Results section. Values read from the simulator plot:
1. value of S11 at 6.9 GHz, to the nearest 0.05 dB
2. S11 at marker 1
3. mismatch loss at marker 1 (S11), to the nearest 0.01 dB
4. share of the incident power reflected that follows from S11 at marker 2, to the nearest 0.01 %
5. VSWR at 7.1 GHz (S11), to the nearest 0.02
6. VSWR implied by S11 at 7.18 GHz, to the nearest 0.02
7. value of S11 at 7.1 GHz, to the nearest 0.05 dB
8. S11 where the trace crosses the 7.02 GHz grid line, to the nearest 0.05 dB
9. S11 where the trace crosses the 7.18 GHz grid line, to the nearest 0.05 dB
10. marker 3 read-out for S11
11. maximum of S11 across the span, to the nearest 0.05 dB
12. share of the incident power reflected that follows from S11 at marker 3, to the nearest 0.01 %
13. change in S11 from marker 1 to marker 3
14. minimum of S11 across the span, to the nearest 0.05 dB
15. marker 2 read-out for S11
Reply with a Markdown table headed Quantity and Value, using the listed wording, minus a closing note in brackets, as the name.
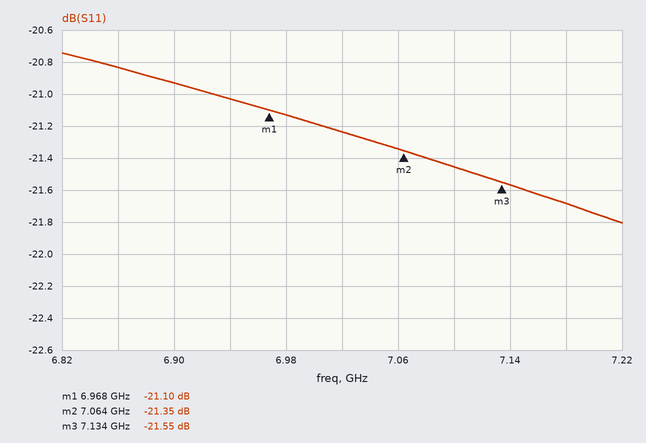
| Quantity | Value |
|---|---|
| value of S11 at 6.9 GHz, to the nearest 0.05 dB | -20.95 dB |
| S11 at marker 1 | -21.10 dB |
| mismatch loss at marker 1 (S11), to the nearest 0.01 dB | 0.03 dB |
| share of the incident power reflected that follows from S11 at marker 2, to the nearest 0.01 % | 0.73 % |
| VSWR at 7.1 GHz (S11), to the nearest 0.02 | 1.18 |
| VSWR implied by S11 at 7.18 GHz, to the nearest 0.02 | 1.18 |
| value of S11 at 7.1 GHz, to the nearest 0.05 dB | -21.45 dB |
| S11 where the trace crosses the 7.02 GHz grid line, to the nearest 0.05 dB | -21.25 dB |
| S11 where the trace crosses the 7.18 GHz grid line, to the nearest 0.05 dB | -21.70 dB |
| marker 3 read-out for S11 | -21.55 dB |
| maximum of S11 across the span, to the nearest 0.05 dB | -20.75 dB |
| share of the incident power reflected that follows from S11 at marker 3, to the nearest 0.01 % | 0.70 % |
| change in S11 from marker 1 to marker 3 | -0.45 dB |
| minimum of S11 across the span, to the nearest 0.05 dB | -21.80 dB |
| marker 2 read-out for S11 | -21.35 dB |
